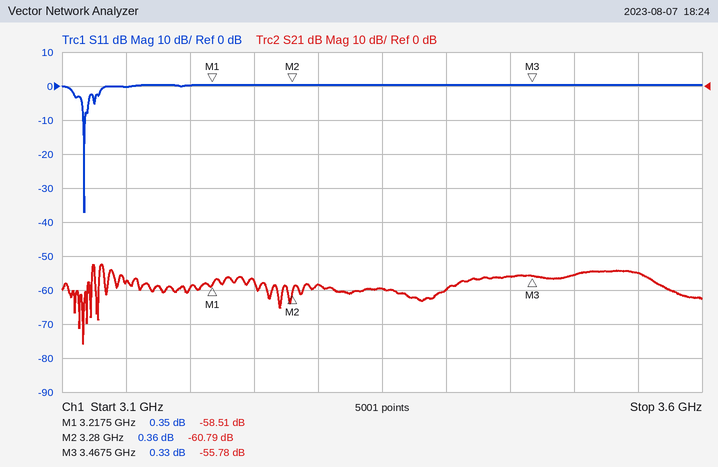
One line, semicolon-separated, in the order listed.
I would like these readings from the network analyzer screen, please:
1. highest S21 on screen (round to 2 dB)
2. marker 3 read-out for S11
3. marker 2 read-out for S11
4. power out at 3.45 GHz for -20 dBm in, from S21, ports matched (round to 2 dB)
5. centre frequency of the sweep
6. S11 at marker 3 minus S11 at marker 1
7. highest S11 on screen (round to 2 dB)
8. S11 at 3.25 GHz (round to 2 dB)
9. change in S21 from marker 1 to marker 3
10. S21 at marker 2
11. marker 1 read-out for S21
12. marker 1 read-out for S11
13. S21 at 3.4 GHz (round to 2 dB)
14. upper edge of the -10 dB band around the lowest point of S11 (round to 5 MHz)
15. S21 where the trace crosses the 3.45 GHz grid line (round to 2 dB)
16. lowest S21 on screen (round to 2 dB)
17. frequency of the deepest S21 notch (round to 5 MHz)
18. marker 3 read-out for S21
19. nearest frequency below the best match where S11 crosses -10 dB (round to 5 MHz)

-52 dB; 0.33 dB; 0.36 dB; -76 dBm; 3.35 GHz; -0.02 dB; 0 dB; 0 dB; 2.73 dB; -60.79 dB; -58.51 dB; 0.35 dB; -60 dB; 3.120 GHz; -56 dB; -76 dB; 3.115 GHz; -55.78 dB; 3.115 GHz
